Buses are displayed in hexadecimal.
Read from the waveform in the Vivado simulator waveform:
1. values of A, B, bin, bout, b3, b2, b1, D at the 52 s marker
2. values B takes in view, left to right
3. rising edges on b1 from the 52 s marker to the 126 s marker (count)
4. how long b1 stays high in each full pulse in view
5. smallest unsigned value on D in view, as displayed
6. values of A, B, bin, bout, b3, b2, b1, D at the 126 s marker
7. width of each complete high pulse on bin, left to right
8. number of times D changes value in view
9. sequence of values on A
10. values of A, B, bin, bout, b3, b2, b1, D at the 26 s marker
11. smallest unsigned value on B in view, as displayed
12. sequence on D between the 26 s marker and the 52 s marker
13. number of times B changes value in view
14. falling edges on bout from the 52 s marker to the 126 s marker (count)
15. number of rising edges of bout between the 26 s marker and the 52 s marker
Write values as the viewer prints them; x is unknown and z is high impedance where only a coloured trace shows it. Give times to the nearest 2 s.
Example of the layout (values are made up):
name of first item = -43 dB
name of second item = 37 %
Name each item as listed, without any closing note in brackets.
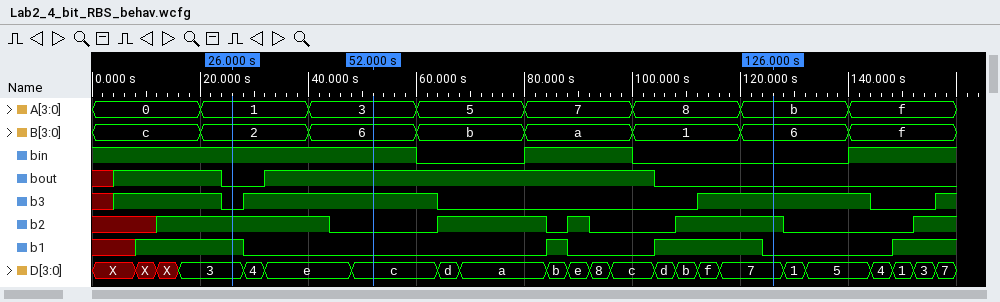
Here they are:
values of A, B, bin, bout, b3, b2, b1, D at the 52 s marker = A=3, B=6, bin=1, bout=1, b3=1, b2=0, b1=0, D=c
values B takes in view, left to right = c, 2, 6, b, a, 1, 6, f
rising edges on b1 from the 52 s marker to the 126 s marker = 2
how long b1 stays high in each full pulse in view = 4 s, 20 s
smallest unsigned value on D in view, as displayed = 1
values of A, B, bin, bout, b3, b2, b1, D at the 126 s marker = A=b, B=6, bin=0, bout=0, b3=1, b2=1, b1=0, D=7
width of each complete high pulse on bin, left to right = 20 s
number of times D changes value in view = 22
sequence of values on A = 0, 1, 3, 5, 7, 8, b, f
values of A, B, bin, bout, b3, b2, b1, D at the 26 s marker = A=1, B=2, bin=1, bout=0, b3=0, b2=1, b1=1, D=3
smallest unsigned value on B in view, as displayed = 1
sequence on D between the 26 s marker and the 52 s marker = 3, 4, e, c
number of times B changes value in view = 7
falling edges on bout from the 52 s marker to the 126 s marker = 1
number of rising edges of bout between the 26 s marker and the 52 s marker = 1
